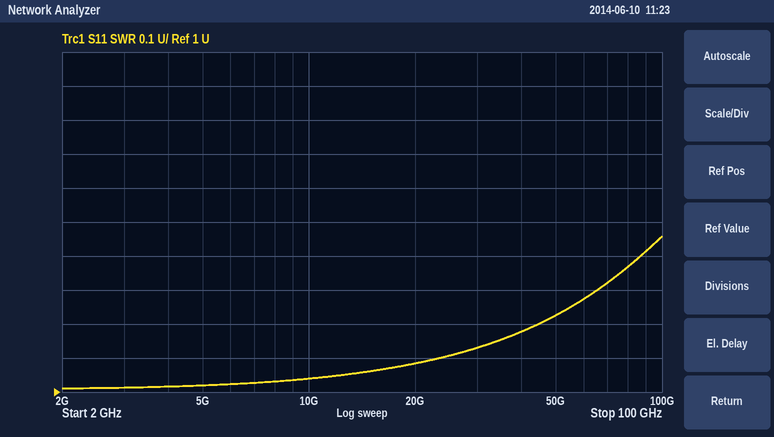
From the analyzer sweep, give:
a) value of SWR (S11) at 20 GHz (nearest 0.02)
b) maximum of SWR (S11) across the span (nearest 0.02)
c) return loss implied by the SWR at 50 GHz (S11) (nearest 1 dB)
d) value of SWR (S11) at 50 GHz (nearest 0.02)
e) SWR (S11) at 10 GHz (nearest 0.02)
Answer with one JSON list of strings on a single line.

["1.08", "1.46", "20 dB", "1.22", "1.04"]
